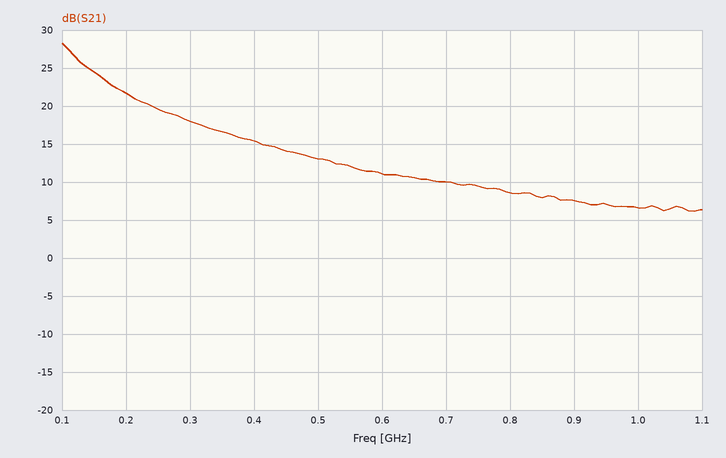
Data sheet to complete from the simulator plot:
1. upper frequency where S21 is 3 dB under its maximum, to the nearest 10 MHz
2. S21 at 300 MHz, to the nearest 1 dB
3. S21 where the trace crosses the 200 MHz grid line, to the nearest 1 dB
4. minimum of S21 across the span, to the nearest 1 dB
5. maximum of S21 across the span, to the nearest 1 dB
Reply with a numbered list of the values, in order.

1. 140 MHz
2. 18 dB
3. 22 dB
4. 6 dB
5. 28 dB
